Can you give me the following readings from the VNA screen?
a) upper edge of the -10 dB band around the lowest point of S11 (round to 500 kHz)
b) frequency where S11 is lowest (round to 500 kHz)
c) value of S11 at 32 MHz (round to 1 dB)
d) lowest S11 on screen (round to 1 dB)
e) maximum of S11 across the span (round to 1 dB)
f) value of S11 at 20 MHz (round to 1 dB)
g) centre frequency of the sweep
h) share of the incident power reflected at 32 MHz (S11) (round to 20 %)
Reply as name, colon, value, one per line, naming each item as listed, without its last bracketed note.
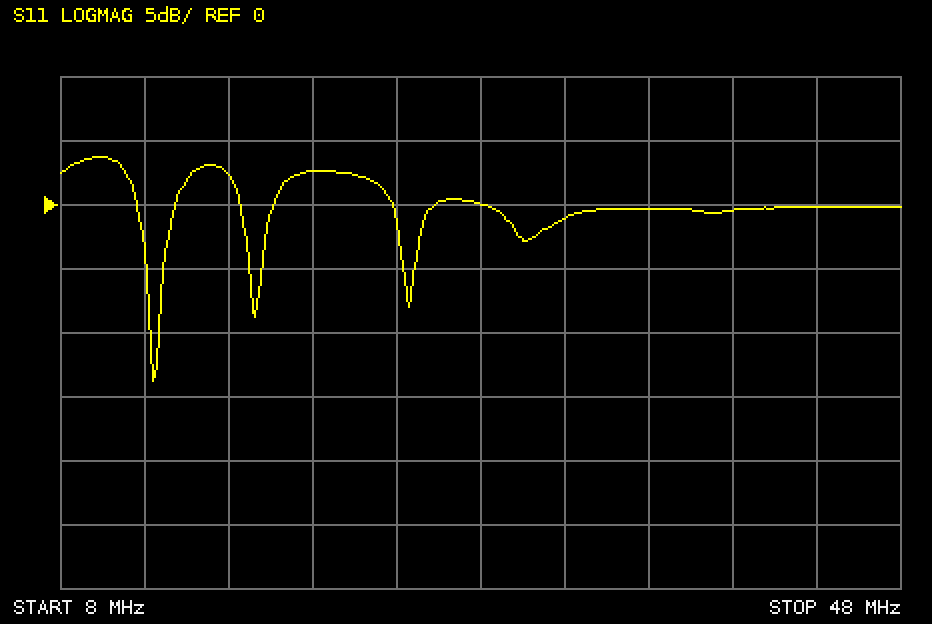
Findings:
upper edge of the -10 dB band around the lowest point of S11: 12.5 MHz
frequency where S11 is lowest: 12.5 MHz
value of S11 at 32 MHz: -1 dB
lowest S11 on screen: -14 dB
maximum of S11 across the span: 4 dB
value of S11 at 20 MHz: 3 dB
centre frequency of the sweep: 28 MHz
share of the incident power reflected at 32 MHz (S11): 80 %
